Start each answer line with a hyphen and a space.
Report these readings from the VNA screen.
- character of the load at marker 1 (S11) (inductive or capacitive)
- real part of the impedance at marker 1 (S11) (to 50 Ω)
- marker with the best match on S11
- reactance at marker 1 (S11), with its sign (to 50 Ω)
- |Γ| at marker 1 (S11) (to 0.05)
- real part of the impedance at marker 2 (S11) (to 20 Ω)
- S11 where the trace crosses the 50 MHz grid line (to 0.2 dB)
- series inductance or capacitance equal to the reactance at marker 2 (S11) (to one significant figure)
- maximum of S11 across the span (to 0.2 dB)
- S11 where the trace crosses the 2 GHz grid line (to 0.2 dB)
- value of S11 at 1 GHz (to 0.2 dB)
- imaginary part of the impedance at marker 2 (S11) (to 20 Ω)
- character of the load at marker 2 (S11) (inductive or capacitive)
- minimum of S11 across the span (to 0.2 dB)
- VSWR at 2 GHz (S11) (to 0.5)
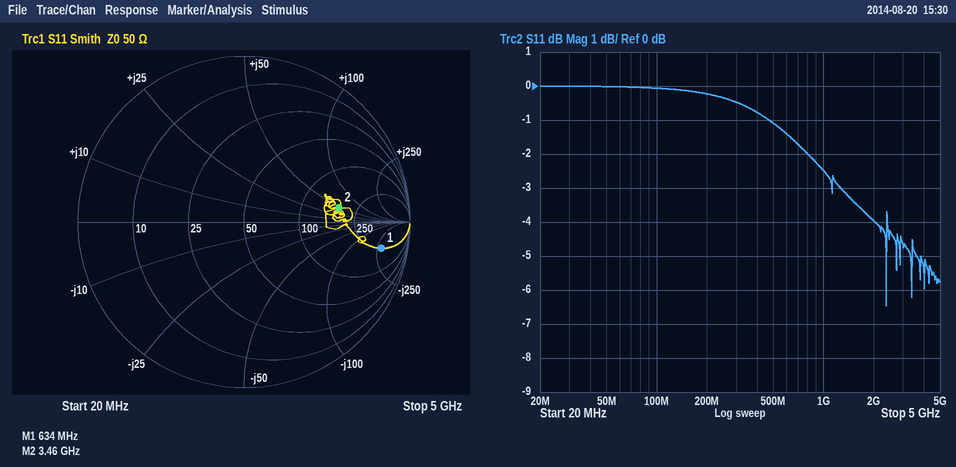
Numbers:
- capacitive
- 250 Ω
- marker 2
- -300 Ω
- 0.85
- 180 Ω
- 0.0 dB
- 2 nH
- 0.0 dB
- -4.0 dB
- -2.4 dB
- +40 Ω
- inductive
- -6.4 dB
- 4.5
